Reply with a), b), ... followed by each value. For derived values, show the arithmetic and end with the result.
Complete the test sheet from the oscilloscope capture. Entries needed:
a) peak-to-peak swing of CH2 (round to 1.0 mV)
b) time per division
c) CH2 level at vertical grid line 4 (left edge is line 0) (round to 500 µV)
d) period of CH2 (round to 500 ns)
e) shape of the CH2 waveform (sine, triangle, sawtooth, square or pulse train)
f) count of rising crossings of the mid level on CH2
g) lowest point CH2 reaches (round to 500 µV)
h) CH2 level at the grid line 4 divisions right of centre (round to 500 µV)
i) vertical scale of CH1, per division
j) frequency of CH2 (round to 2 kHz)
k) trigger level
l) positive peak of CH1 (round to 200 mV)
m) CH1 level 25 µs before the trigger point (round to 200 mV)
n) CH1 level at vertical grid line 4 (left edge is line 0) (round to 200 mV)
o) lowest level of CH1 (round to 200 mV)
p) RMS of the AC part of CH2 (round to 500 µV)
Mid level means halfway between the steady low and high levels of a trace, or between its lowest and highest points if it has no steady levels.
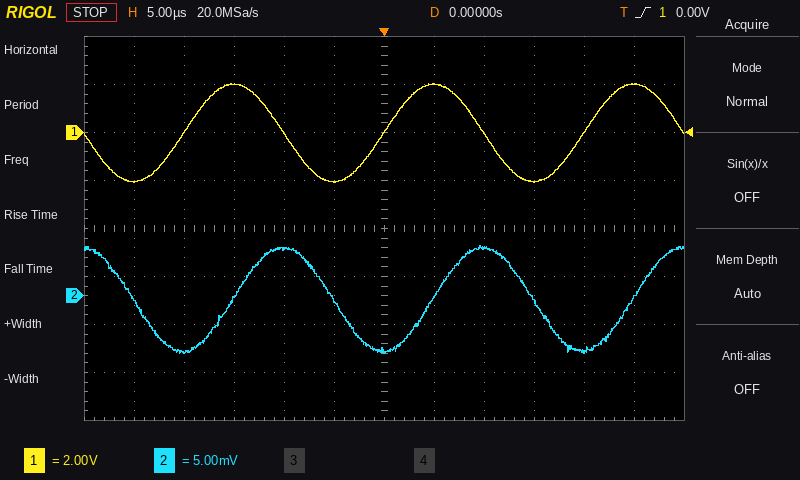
a) 11.0 mV
b) 5 µs
c) 5.0 mV
d) 20.0 µs
e) sine
f) 3
g) -6.0 mV
h) -5.5 mV
i) 2 V
j) 1 / 20.0 µs ≈ 50 kHz
k) 0.00 V
l) 2.0 V
m) -2.0 V
n) 0.0 V
o) -2.0 V
p) 11.0 mV / (2√2) ≈ 3.89 mV, so 4.0 mV to the nearest 500 µV
